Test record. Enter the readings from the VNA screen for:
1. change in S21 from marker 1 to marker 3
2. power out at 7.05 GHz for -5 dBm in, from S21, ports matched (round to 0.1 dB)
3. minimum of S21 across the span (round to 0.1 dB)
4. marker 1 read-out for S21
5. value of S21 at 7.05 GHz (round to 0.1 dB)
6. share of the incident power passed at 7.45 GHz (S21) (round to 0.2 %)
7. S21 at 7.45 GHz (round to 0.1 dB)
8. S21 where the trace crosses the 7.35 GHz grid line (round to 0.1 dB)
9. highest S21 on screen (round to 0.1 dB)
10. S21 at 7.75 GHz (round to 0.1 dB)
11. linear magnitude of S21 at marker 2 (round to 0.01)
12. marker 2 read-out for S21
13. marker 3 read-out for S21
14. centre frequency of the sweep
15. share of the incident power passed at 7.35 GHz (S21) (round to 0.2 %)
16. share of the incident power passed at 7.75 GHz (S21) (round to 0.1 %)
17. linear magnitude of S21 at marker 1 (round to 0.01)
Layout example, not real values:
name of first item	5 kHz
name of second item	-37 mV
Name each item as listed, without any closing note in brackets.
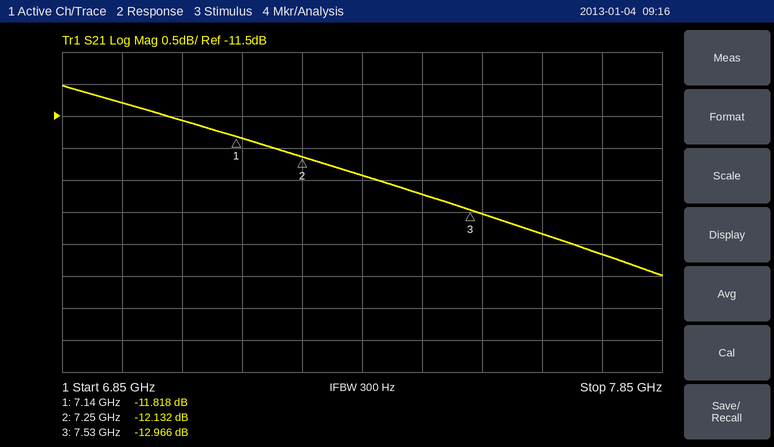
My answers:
change in S21 from marker 1 to marker 3	-1.148 dB
power out at 7.05 GHz for -5 dBm in, from S21, ports matched	-16.6 dBm
minimum of S21 across the span	-14.0 dB
marker 1 read-out for S21	-11.818 dB
value of S21 at 7.05 GHz	-11.6 dB
share of the incident power passed at 7.45 GHz (S21)	5.4 %
S21 at 7.45 GHz	-12.7 dB
S21 where the trace crosses the 7.35 GHz grid line	-12.4 dB
highest S21 on screen	-11.0 dB
S21 at 7.75 GHz	-13.7 dB
linear magnitude of S21 at marker 2	0.25
marker 2 read-out for S21	-12.132 dB
marker 3 read-out for S21	-12.966 dB
centre frequency of the sweep	7.35 GHz
share of the incident power passed at 7.35 GHz (S21)	5.8 %
share of the incident power passed at 7.75 GHz (S21)	4.3 %
linear magnitude of S21 at marker 1	0.26
